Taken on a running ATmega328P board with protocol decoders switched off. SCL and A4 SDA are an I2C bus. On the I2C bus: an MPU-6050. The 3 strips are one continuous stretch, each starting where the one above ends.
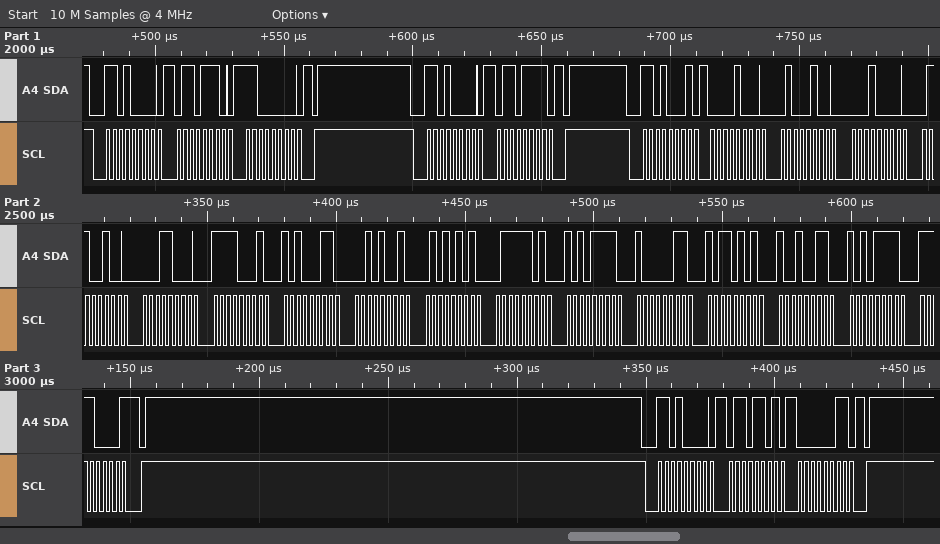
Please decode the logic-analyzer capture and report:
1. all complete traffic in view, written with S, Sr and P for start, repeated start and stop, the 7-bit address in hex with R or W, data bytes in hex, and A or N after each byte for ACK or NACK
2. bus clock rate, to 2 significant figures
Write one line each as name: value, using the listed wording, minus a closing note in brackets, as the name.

all complete traffic in view, written with S, Sr and P for start, repeated start and stop, the 7-bit address in hex with R or W, data bytes in hex, and A or N after each byte for ACK or NACK: S 68W A 6E A C0 A P S 68W A 6F A P S 68R A 08 A 44 A 10 A 64 A 18 A F1 A A3 A 29 A 55 A 7D A AF A 83 A B5 A 93 A AF A F0 N P S 68W A 6D A 03 A P
bus clock rate, to 2 significant figures: 400 kHz
